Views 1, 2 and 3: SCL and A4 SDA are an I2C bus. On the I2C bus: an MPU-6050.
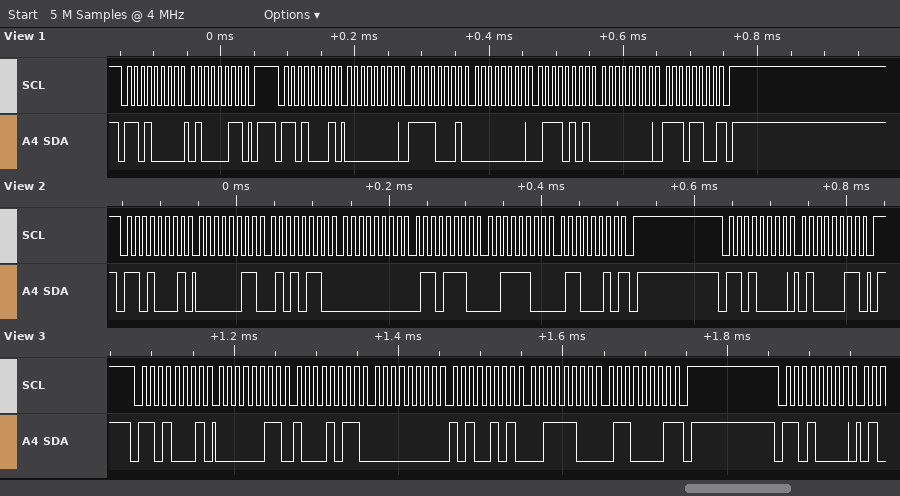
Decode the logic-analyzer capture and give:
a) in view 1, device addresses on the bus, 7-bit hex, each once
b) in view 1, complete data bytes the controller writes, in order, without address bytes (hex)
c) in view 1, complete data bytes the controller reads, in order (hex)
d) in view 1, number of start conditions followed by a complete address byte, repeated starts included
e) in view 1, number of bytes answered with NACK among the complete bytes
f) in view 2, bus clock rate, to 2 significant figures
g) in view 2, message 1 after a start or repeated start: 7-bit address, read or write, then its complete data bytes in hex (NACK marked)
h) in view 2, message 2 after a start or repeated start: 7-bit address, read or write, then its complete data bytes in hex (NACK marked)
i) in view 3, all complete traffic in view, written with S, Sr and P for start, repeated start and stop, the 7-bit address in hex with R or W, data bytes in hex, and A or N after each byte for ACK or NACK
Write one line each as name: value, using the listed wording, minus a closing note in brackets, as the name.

in view 1, device addresses on the bus, 7-bit hex, each once: 0x68
in view 1, complete data bytes the controller writes, in order, without address bytes: 43
in view 1, complete data bytes the controller reads, in order: 00 F1 00 75 00 EC
in view 1, number of start conditions followed by a complete address byte, repeated starts included: 2
in view 1, number of bytes answered with NACK among the complete bytes: 1
in view 2, bus clock rate, to 2 significant figures: 100 kHz
in view 2, message 1 after a start or repeated start: 7-bit address, read or write, then its complete data bytes in hex: 0x68 read: 03 56 00 6E 3C 62 NACK
in view 2, message 2 after a start or repeated start: 7-bit address, read or write, then its complete data bytes in hex: 0x68 write: 43
in view 3, all complete traffic in view, written with S, Sr and P for start, repeated start and stop, the 7-bit address in hex with R or W, data bytes in hex, and A or N after each byte for ACK or NACK: S 68R A 03 A 8B A 00 A A5 A 3C A 61 N P S 68W A
